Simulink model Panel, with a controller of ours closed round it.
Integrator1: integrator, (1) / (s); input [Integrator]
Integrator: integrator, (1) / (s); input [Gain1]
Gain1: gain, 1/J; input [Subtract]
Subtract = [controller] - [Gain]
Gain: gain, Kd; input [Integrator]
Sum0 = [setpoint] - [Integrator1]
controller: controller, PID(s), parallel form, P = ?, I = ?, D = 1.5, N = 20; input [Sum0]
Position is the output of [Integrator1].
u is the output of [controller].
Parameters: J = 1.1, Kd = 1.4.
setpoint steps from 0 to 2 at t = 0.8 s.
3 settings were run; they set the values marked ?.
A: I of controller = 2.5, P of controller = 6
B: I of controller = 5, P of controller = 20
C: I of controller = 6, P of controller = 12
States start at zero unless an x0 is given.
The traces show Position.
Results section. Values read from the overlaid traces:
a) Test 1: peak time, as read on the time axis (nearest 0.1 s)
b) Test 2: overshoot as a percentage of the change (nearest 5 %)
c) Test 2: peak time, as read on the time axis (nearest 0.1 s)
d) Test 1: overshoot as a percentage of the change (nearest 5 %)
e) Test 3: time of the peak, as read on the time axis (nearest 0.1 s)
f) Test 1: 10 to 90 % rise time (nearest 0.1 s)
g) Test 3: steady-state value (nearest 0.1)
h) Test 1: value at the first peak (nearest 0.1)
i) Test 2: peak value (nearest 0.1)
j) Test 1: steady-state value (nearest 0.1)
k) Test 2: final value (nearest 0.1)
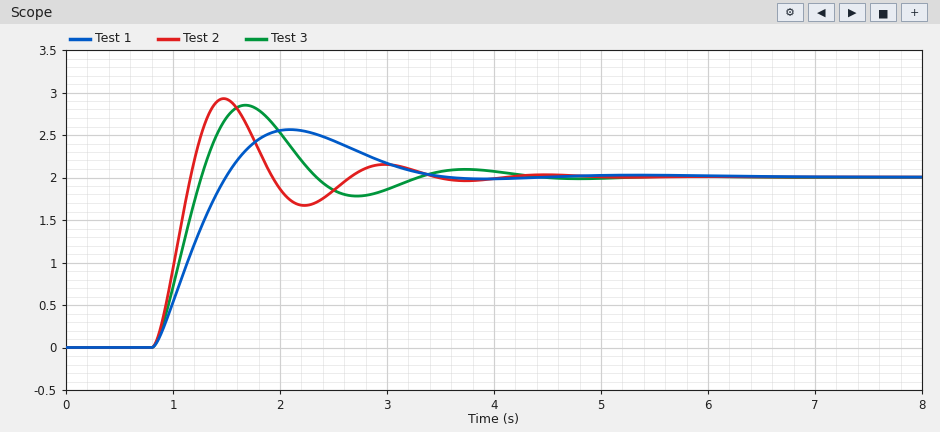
2.1 s
45 %
1.5 s
30 %
1.7 s
0.5 s
2.0
2.6
2.9
2.0
2.0
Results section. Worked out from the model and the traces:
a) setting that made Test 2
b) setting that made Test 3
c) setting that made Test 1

B
C
A
